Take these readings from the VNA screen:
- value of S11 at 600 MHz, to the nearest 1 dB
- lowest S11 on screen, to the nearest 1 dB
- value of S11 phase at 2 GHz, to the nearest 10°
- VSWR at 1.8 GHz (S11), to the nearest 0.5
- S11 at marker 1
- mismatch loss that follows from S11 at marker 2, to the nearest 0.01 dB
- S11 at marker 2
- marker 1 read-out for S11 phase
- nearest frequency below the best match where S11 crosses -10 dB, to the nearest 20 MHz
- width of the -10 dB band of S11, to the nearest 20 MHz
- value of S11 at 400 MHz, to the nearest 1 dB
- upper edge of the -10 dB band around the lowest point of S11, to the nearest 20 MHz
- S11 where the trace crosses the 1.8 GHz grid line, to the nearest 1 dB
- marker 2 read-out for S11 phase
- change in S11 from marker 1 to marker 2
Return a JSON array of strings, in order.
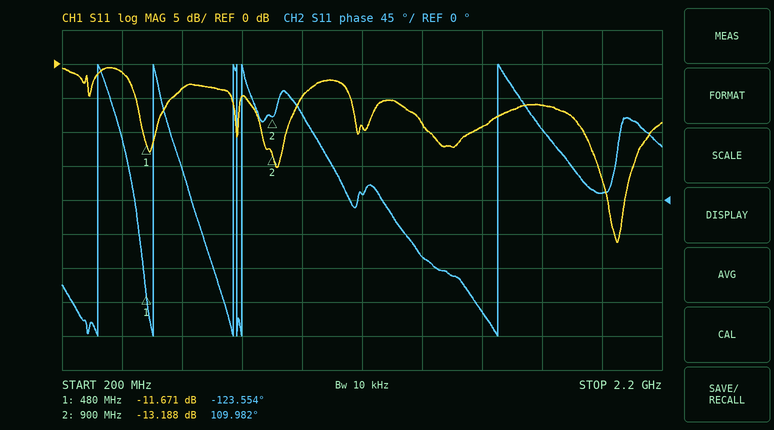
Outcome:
["-4 dB", "-26 dB", "10°", "3.0", "-11.671 dB", "0.21 dB", "-13.188 dB", "-123.554°", "1.94 GHz", "220 MHz", "-1 dB", "2.16 GHz", "-6 dB", "109.982°", "-1.517 dB"]
